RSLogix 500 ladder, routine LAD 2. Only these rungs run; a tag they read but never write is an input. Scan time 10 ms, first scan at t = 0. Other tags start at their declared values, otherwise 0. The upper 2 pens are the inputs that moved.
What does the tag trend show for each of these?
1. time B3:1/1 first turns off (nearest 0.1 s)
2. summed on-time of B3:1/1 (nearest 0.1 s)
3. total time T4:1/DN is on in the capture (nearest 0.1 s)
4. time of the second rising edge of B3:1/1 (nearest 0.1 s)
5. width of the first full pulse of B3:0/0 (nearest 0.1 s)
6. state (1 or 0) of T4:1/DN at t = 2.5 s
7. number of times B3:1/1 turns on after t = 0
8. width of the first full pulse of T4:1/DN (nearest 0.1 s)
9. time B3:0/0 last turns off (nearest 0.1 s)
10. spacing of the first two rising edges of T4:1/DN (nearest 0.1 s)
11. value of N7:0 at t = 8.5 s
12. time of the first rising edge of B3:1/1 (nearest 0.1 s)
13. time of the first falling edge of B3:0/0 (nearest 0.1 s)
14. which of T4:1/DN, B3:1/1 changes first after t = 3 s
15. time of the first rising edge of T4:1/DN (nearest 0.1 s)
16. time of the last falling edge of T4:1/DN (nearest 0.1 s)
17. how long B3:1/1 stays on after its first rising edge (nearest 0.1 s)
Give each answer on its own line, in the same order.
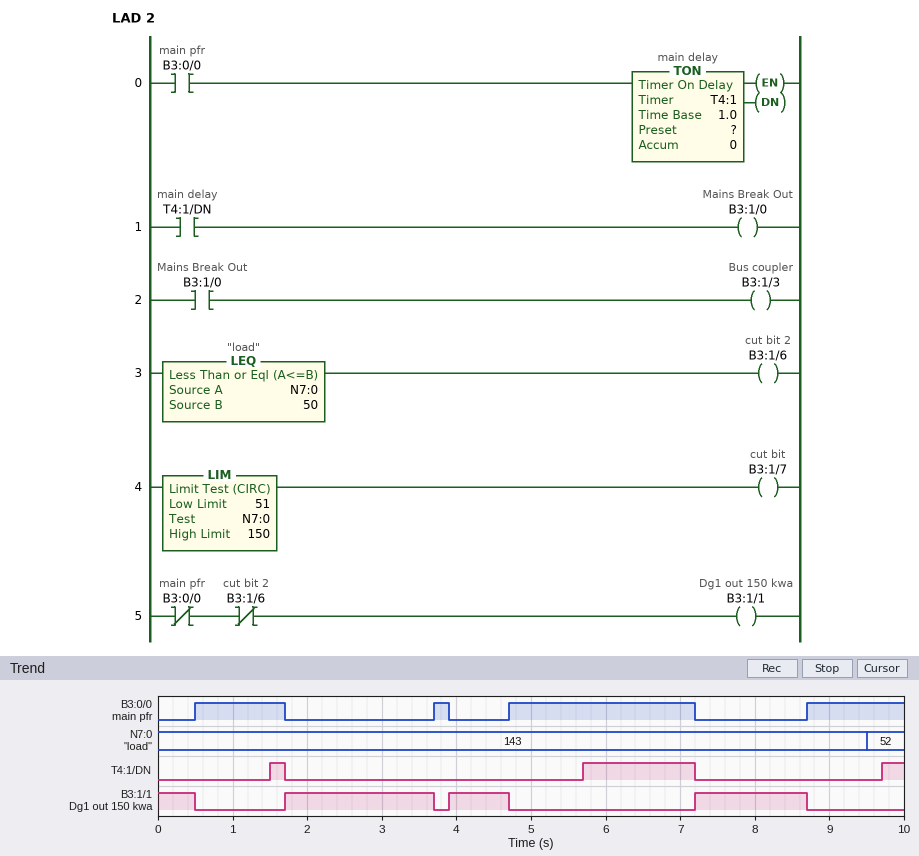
0.5 s
4.8 s
2.0 s
3.9 s
1.2 s
0
3
0.2 s
7.2 s
4.2 s
143
1.7 s
1.7 s
B3:1/1
1.5 s
7.2 s
2.0 s
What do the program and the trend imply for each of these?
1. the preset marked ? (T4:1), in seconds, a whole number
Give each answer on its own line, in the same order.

1 s
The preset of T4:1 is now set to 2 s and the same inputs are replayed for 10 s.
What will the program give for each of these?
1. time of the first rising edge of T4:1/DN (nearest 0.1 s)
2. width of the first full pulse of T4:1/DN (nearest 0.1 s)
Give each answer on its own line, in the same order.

6.7 s
0.5 s
